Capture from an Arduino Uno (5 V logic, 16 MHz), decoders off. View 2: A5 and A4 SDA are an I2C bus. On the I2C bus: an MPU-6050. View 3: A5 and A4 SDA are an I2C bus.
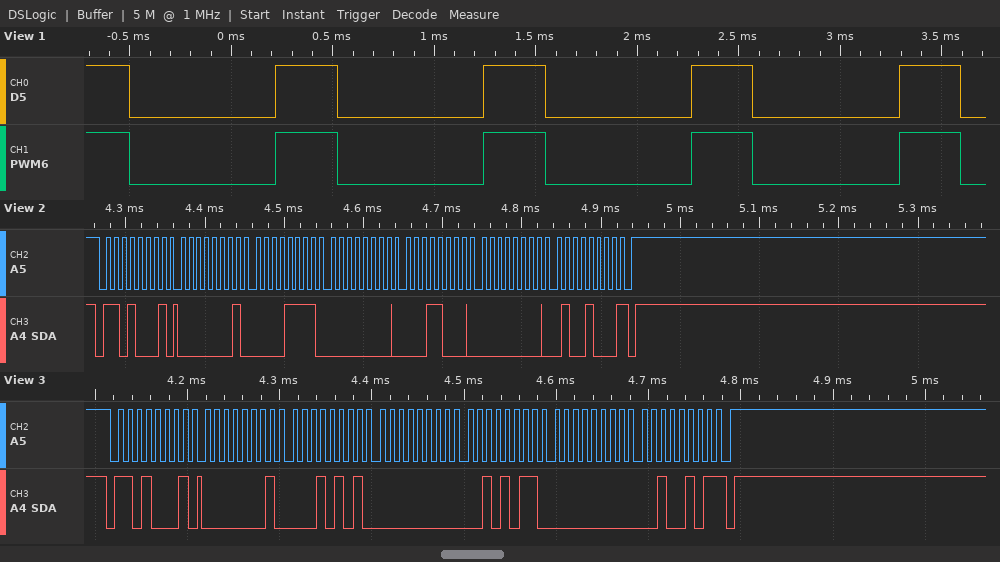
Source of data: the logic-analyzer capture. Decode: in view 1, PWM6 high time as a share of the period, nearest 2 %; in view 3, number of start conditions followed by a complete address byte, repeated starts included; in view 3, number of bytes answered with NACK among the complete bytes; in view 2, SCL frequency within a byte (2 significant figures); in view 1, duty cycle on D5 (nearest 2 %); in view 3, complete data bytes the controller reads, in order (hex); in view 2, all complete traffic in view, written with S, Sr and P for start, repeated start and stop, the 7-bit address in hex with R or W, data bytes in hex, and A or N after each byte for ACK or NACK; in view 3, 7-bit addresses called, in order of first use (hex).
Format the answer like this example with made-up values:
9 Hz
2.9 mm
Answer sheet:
30 %
1
1
100 kHz
30 %
01 15 00 2B 00 25
S 68R A 01 A 0F A 00 A 18 A 00 A 48 N P
0x68
